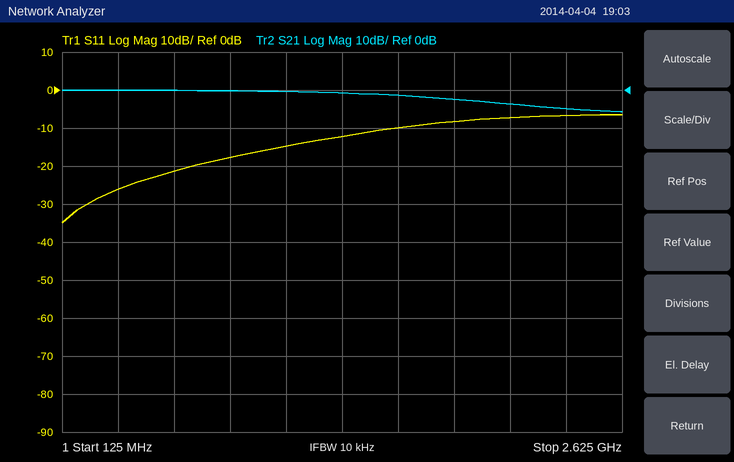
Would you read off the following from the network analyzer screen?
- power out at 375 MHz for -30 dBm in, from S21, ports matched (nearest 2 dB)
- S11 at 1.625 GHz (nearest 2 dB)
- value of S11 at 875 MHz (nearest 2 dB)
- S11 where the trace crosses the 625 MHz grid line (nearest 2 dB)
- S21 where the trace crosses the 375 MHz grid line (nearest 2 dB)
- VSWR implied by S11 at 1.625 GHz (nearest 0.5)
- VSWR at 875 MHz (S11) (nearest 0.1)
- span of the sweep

-30 dBm
-10 dB
-18 dB
-22 dB
0 dB
2.0
1.3
2.5 GHz
